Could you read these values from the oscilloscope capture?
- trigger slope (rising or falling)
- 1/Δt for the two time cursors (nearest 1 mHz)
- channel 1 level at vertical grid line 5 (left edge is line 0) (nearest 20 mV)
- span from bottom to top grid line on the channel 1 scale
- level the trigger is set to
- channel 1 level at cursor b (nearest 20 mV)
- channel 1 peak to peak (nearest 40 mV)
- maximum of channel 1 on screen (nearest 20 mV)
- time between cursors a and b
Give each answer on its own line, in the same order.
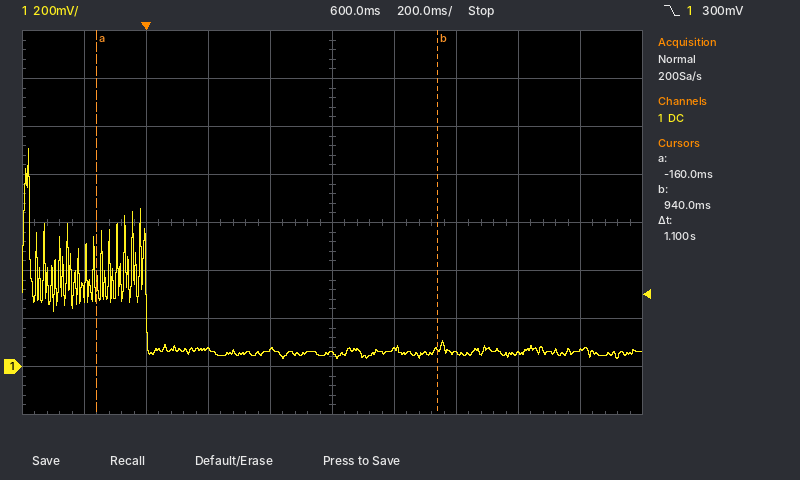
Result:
falling
909 mHz
60 mV
1.6 V
300 mV
80 mV
880 mV
900 mV
1.1 s
